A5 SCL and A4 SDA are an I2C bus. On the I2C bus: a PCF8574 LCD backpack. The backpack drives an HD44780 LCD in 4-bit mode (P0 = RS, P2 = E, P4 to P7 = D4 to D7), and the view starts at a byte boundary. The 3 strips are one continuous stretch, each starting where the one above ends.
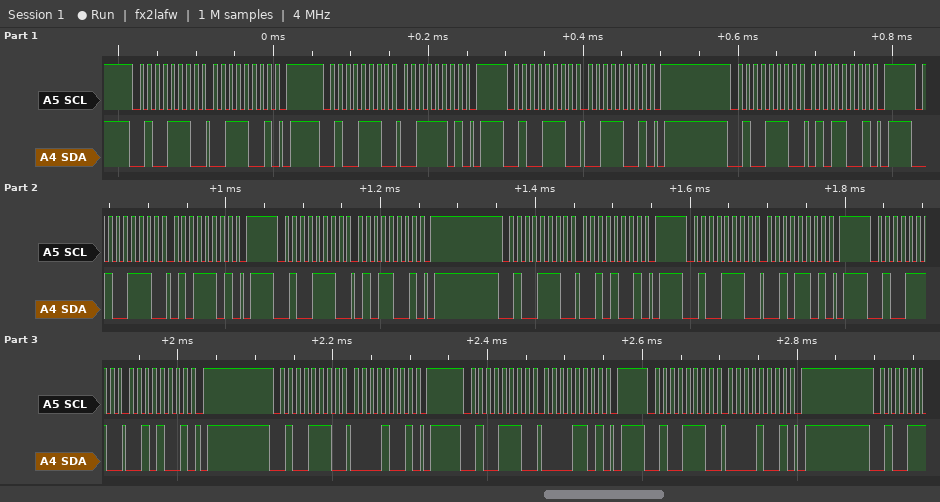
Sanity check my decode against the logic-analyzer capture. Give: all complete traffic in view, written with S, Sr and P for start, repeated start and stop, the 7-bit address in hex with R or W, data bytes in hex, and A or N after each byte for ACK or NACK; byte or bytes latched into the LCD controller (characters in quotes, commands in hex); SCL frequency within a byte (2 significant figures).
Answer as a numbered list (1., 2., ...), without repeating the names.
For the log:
1. S 27W A 39 A P S 27W A 3D A P S 27W A 39 A P S 27W A 59 A P S 27W A 5D A P S 27W A 59 A P S 27W A 29 A P S 27W A 2D A P S 27W A 29 A P S 27W A 09 A P S 27W A 0D A P S 27W A 09 A P
2. '5' ' '
3. 100 kHz
